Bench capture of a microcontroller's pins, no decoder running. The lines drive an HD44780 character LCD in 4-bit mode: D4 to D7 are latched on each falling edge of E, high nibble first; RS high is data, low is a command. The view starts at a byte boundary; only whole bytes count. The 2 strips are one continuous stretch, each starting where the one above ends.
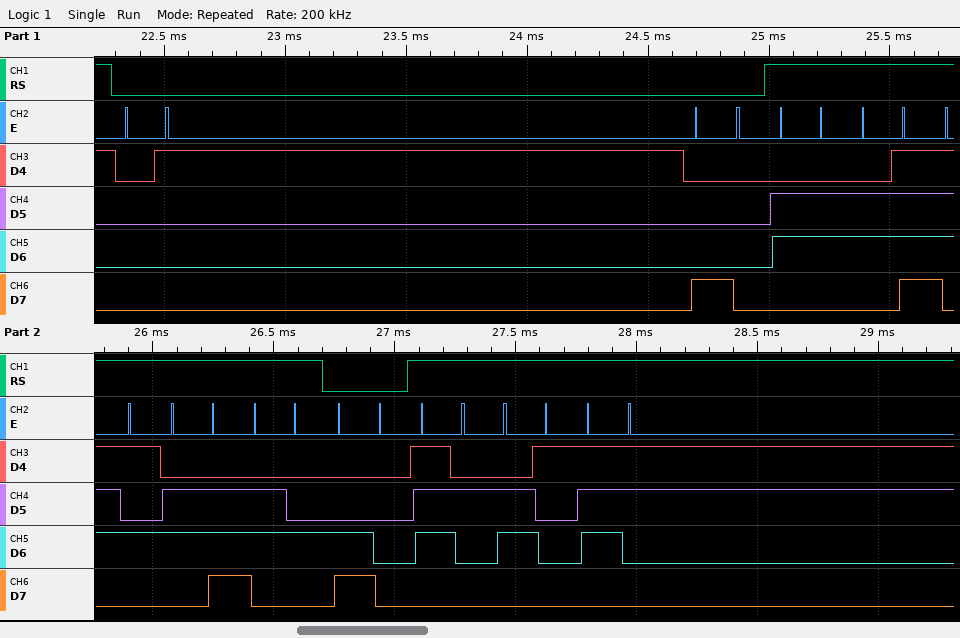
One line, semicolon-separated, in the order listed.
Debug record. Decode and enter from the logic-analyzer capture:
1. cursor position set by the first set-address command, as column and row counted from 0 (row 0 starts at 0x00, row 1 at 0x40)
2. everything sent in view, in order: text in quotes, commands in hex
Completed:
column 0, row 0; 0x01 0x80 "found" 0xC0 "ras"
